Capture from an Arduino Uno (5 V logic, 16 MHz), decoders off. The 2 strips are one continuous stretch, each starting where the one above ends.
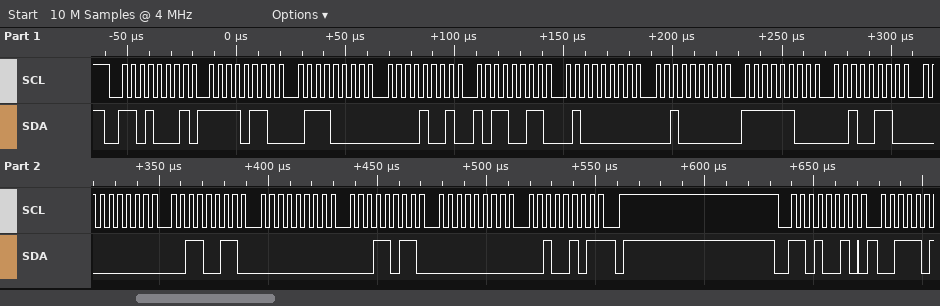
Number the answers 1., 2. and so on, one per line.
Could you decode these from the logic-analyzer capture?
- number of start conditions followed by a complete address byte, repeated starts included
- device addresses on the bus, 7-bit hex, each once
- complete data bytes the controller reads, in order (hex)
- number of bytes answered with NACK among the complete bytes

1. 2
2. 0x68 0x69
3. F6 70 09 B3 40 20 FC 26 00 33 00 1B 00 25
4. 1
